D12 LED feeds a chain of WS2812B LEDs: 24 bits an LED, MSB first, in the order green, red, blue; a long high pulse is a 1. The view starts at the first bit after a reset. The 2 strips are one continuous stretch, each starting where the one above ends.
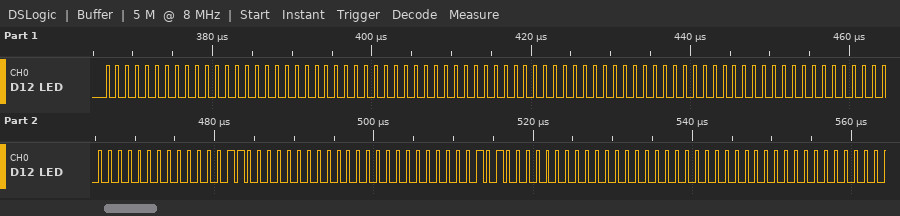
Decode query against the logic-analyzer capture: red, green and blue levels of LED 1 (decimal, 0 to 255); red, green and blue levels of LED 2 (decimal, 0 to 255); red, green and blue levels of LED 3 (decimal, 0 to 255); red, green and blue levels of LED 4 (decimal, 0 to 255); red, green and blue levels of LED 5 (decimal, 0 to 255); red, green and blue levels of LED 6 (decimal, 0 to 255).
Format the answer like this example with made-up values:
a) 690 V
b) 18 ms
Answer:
a) 0, 0, 0
b) 0, 0, 0
c) 0, 0, 0
d) 0, 0, 12
e) 0, 0, 5
f) 0, 0, 0
